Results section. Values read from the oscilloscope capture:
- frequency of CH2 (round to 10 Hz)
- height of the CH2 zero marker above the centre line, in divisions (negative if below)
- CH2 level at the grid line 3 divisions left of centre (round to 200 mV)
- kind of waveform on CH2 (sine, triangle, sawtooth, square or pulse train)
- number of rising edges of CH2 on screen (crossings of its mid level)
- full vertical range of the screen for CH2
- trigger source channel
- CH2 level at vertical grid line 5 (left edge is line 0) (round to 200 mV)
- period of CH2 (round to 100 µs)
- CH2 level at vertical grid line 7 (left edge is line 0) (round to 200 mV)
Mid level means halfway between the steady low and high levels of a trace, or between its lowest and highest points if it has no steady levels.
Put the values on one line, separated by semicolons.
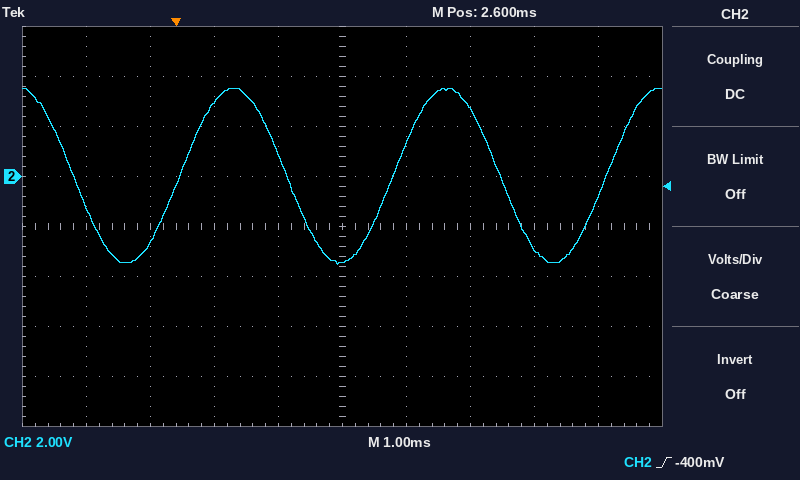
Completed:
300 Hz; +1.0 div; -2.6 V; sine; 3; 16 V; CH2; -3.4 V; 3.3 ms; 2.8 V
